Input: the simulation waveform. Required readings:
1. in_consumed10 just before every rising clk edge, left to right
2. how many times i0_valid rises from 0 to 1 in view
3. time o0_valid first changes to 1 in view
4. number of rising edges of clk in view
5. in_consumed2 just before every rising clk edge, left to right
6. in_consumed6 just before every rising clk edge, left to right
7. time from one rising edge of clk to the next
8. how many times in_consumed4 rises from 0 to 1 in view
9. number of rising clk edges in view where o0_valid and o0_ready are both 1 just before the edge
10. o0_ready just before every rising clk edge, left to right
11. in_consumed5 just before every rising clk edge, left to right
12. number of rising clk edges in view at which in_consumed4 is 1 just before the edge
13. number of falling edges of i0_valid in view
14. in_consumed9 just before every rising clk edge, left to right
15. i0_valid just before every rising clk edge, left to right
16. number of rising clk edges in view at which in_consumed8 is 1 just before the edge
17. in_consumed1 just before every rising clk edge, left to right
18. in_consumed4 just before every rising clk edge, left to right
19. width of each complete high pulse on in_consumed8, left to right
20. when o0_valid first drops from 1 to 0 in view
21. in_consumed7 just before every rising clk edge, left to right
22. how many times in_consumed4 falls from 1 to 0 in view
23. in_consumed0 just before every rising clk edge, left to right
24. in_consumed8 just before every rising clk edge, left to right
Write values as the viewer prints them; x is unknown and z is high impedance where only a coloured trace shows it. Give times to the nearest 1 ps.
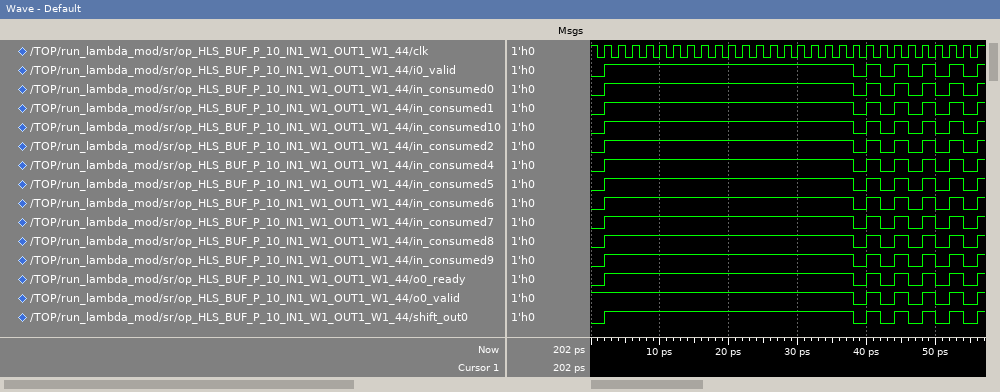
0 1 1 1 1 1 1 1 1 1 1 1 1 1 1 1 1 1 1 0 1 0 1 0 1 0 1 0
6
40 ps
28
0 1 1 1 1 1 1 1 1 1 1 1 1 1 1 1 1 1 1 0 1 0 1 0 1 0 1 0
0 1 1 1 1 1 1 1 1 1 1 1 1 1 1 1 1 1 1 0 1 0 1 0 1 0 1 0
2 ps
6
22
0 1 1 1 1 1 1 1 1 1 1 1 1 1 1 1 1 1 1 0 1 0 1 0 1 0 1 0
0 1 1 1 1 1 1 1 1 1 1 1 1 1 1 1 1 1 1 0 1 0 1 0 1 0 1 0
22
5
0 1 1 1 1 1 1 1 1 1 1 1 1 1 1 1 1 1 1 0 1 0 1 0 1 0 1 0
0 1 1 1 1 1 1 1 1 1 1 1 1 1 1 1 1 1 1 0 1 0 1 0 1 0 1 0
22
0 1 1 1 1 1 1 1 1 1 1 1 1 1 1 1 1 1 1 0 1 0 1 0 1 0 1 0
0 1 1 1 1 1 1 1 1 1 1 1 1 1 1 1 1 1 1 0 1 0 1 0 1 0 1 0
36 ps, 2 ps, 2 ps, 2 ps, 2 ps
38 ps
0 1 1 1 1 1 1 1 1 1 1 1 1 1 1 1 1 1 1 0 1 0 1 0 1 0 1 0
5
0 1 1 1 1 1 1 1 1 1 1 1 1 1 1 1 1 1 1 0 1 0 1 0 1 0 1 0
0 1 1 1 1 1 1 1 1 1 1 1 1 1 1 1 1 1 1 0 1 0 1 0 1 0 1 0
